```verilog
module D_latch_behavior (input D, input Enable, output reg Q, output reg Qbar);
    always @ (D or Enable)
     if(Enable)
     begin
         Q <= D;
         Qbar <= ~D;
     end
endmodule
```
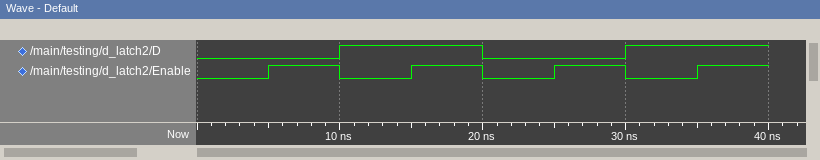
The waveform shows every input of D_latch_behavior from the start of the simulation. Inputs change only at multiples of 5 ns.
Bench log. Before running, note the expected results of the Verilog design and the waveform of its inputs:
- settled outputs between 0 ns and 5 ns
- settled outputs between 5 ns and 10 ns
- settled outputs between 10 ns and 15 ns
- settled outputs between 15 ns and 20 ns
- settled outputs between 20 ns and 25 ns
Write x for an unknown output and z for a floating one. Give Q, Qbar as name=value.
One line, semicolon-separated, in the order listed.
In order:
Q=x, Qbar=x; Q=0, Qbar=1; Q=0, Qbar=1; Q=1, Qbar=0; Q=1, Qbar=0
